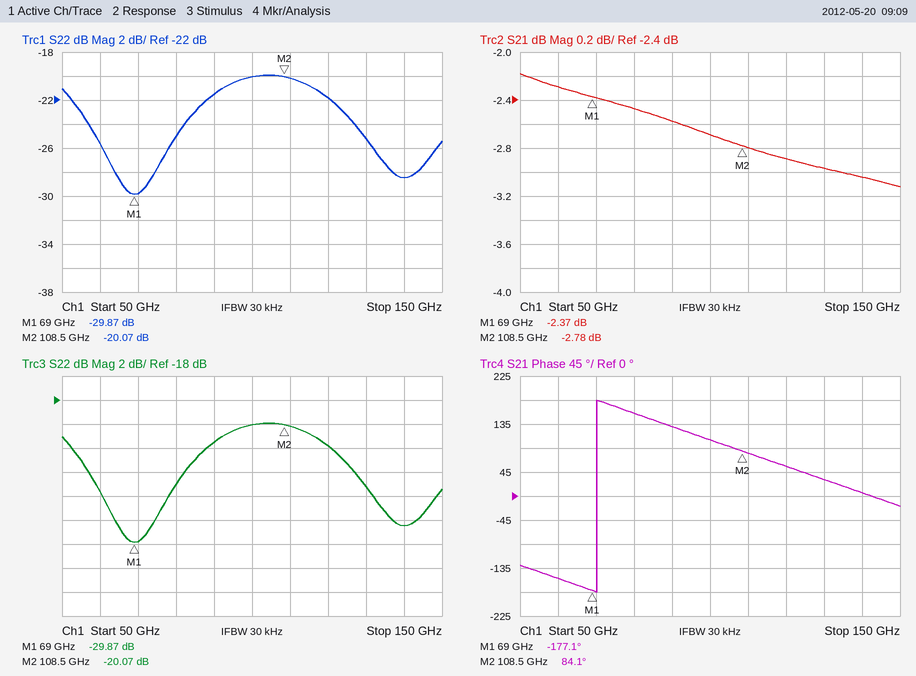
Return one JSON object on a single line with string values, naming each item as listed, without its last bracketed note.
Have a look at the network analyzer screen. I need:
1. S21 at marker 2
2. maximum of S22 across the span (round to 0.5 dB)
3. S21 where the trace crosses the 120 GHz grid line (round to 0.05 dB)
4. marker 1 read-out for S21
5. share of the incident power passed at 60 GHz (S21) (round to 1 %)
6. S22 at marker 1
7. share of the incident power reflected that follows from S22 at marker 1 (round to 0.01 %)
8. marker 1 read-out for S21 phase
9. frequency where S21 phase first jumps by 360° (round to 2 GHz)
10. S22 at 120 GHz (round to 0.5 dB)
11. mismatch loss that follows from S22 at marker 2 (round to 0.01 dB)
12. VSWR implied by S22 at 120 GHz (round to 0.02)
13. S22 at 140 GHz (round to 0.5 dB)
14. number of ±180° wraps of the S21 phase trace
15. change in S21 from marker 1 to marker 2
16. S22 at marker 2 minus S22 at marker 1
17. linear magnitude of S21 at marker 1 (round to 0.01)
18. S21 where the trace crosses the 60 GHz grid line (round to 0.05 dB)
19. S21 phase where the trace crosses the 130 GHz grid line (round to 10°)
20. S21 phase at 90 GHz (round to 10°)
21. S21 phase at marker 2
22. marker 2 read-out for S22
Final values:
{"S21 at marker 2": "-2.78 dB", "maximum of S22 across the span": "-20.0 dB", "S21 where the trace crosses the 120 GHz grid line": "-2.90 dB", "marker 1 read-out for S21": "-2.37 dB", "share of the incident power passed at 60 GHz (S21)": "59 %", "S22 at marker 1": "-29.87 dB", "share of the incident power reflected that follows from S22 at marker 1": "0.10 %", "marker 1 read-out for S21 phase": "-177.1°", "frequency where S21 phase first jumps by 360°": "70 GHz", "S22 at 120 GHz": "-22.0 dB", "mismatch loss that follows from S22 at marker 2": "0.04 dB", "VSWR implied by S22 at 120 GHz": "1.18", "S22 at 140 GHz": "-28.5 dB", "number of ±180° wraps of the S21 phase trace": "1", "change in S21 from marker 1 to marker 2": "-0.41 dB", "S22 at marker 2 minus S22 at marker 1": "9.80 dB", "linear magnitude of S21 at marker 1": "0.76", "S21 where the trace crosses the 60 GHz grid line": "-2.30 dB", "S21 phase where the trace crosses the 130 GHz grid line": "30°", "S21 phase at 90 GHz": "130°", "S21 phase at marker 2": "84.1°", "marker 2 read-out for S22": "-20.07 dB"}
